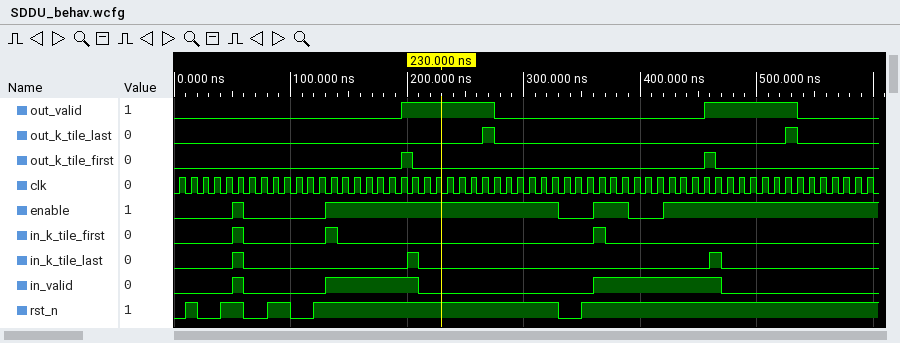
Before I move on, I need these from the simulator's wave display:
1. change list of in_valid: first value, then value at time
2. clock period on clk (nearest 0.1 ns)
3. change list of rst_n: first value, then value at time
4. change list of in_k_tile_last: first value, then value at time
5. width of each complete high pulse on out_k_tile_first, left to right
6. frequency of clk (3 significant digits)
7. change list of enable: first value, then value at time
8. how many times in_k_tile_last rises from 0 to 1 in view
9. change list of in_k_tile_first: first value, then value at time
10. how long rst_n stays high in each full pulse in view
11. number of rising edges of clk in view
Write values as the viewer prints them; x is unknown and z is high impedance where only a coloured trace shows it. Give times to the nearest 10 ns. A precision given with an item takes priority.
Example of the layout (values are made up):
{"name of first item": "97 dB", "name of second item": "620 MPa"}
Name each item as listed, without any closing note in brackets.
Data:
{"change list of in_valid: first value, then value at time": "0, 1 at 50 ns, 0 at 60 ns, 1 at 130 ns, 0 at 210 ns, 1 at 360 ns, 0 at 470 ns", "clock period on clk": "10 ns", "change list of rst_n: first value, then value at time": "0, 1 at 10 ns, 0 at 20 ns, 1 at 40 ns, 0 at 60 ns, 1 at 80 ns, 0 at 100 ns, 1 at 120 ns, 0 at 330 ns, 1 at 350 ns", "change list of in_k_tile_last: first value, then value at time": "0, 1 at 50 ns, 0 at 60 ns, 1 at 200 ns, 0 at 210 ns, 1 at 460 ns, 0 at 470 ns", "width of each complete high pulse on out_k_tile_first, left to right": "10 ns, 10 ns", "frequency of clk": "100 MHz", "change list of enable: first value, then value at time": "0, 1 at 50 ns, 0 at 60 ns, 1 at 130 ns, 0 at 330 ns, 1 at 360 ns, 0 at 390 ns, 1 at 420 ns", "how many times in_k_tile_last rises from 0 to 1 in view": "3", "change list of in_k_tile_first: first value, then value at time": "0, 1 at 50 ns, 0 at 60 ns, 1 at 130 ns, 0 at 140 ns, 1 at 360 ns, 0 at 370 ns", "how long rst_n stays high in each full pulse in view": "10 ns, 20 ns, 20 ns, 210 ns", "number of rising edges of clk in view": "60"}
